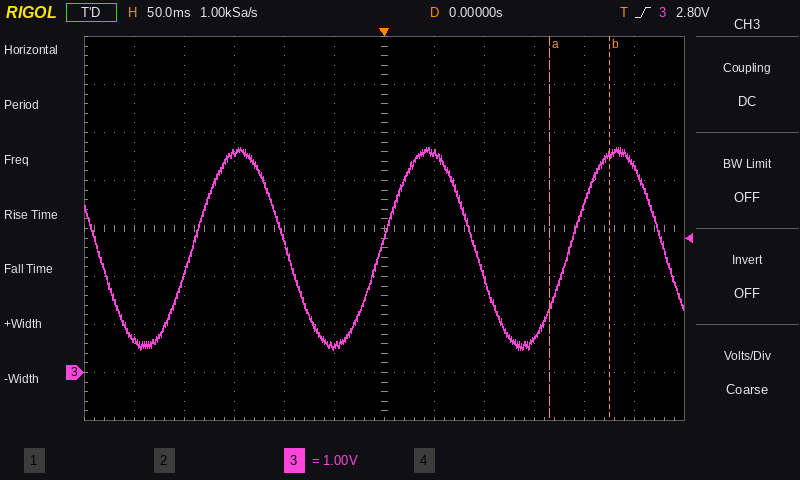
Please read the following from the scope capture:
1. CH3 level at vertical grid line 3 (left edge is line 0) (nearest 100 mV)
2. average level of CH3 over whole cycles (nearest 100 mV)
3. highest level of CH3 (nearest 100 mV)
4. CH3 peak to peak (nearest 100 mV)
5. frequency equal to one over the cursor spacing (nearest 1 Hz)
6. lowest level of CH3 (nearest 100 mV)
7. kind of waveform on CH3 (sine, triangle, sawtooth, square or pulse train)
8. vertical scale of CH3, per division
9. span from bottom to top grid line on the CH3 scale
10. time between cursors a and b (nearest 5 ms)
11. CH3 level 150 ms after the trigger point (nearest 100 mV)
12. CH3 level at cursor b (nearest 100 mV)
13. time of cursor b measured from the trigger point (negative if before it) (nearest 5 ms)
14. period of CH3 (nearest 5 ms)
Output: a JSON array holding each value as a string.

["4.6 V", "2.6 V", "4.7 V", "4.2 V", "17 Hz", "500 mV", "sine", "1 V", "8 V", "60 ms", "700 mV", "4.6 V", "+225 ms", "190 ms"]
